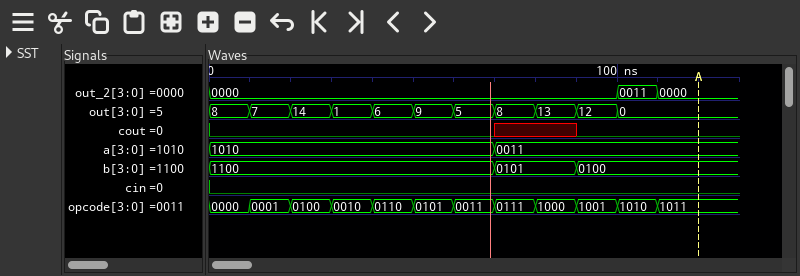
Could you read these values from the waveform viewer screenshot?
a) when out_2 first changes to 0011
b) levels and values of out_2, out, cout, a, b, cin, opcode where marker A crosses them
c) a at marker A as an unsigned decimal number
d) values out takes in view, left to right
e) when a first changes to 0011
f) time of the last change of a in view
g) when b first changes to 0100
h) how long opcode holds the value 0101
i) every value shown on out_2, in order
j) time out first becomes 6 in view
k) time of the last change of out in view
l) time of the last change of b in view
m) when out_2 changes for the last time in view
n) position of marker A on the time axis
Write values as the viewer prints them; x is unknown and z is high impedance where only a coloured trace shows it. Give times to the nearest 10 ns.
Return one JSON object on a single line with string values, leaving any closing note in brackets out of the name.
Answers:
{"when out_2 first changes to 0011": "100 ns", "levels and values of out_2, out, cout, a, b, cin, opcode where marker A crosses them": "out_2=0000, out=0, cout=0, a=0011, b=0100, cin=0, opcode=1011", "a at marker A as an unsigned decimal number": "3", "values out takes in view, left to right": "8, 7, 14, 1, 6, 9, 5, 8, 13, 12, 0", "when a first changes to 0011": "70 ns", "time of the last change of a in view": "70 ns", "when b first changes to 0100": "90 ns", "how long opcode holds the value 0101": "10 ns", "every value shown on out_2, in order": "0000, 0011, 0000", "time out first becomes 6 in view": "40 ns", "time of the last change of out in view": "100 ns", "time of the last change of b in view": "90 ns", "when out_2 changes for the last time in view": "110 ns", "position of marker A on the time axis": "120 ns"}
